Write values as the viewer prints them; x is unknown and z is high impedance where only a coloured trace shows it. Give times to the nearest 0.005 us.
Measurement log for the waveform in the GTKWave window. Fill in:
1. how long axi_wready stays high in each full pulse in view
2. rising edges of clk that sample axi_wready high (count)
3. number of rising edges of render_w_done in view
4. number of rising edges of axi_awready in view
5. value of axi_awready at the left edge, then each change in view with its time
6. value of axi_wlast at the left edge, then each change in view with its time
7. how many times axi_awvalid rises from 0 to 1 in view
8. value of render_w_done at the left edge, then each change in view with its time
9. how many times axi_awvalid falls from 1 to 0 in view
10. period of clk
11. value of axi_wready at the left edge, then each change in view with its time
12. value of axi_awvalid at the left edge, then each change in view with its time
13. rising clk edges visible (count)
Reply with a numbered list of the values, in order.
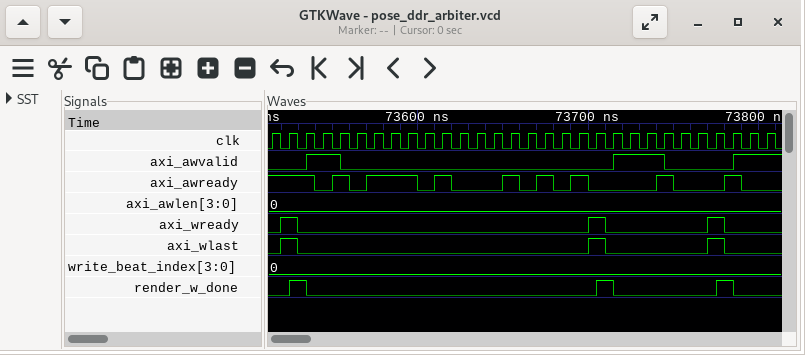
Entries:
1. 0.01 us, 0.01 us, 0.01 us
2. 3
3. 3
4. 8
5. 1, 0 at 73.54 us, 1 at 73.55 us, 0 at 73.56 us, 1 at 73.57 us, 0 at 73.6 us, 1 at 73.61 us, 0 at 73.62 us, 1 at 73.65 us, 0 at 73.66 us, 1 at 73.67 us, 0 at 73.68 us, 1 at 73.69 us, 0 at 73.7 us, 1 at 73.74 us, 0 at 73.75 us, 1 at 73.78 us, 0 at 73.79 us
6. 0, 1 at 73.52 us, 0 at 73.53 us, 1 at 73.7 us, 0 at 73.71 us, 1 at 73.77 us, 0 at 73.78 us
7. 3
8. 0, 1 at 73.525 us, 0 at 73.535 us, 1 at 73.705 us, 0 at 73.715 us, 1 at 73.775 us, 0 at 73.785 us
9. 2
10. 0.01 us
11. 0, 1 at 73.52 us, 0 at 73.53 us, 1 at 73.7 us, 0 at 73.71 us, 1 at 73.77 us, 0 at 73.78 us
12. 0, 1 at 73.535 us, 0 at 73.555 us, 1 at 73.715 us, 0 at 73.745 us, 1 at 73.785 us
13. 30
